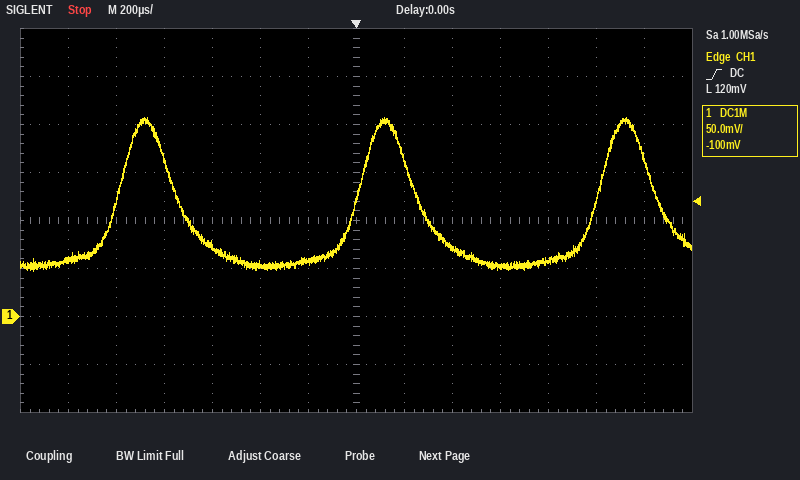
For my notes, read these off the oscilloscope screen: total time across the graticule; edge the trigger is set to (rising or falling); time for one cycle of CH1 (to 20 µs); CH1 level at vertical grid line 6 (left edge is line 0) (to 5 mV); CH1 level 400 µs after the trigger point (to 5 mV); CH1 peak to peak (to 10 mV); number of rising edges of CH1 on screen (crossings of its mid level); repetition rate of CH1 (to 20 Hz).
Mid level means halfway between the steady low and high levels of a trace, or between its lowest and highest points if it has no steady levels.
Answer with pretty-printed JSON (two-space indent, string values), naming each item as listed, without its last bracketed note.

{
  "total time across the graticule": "2.8 ms",
  "edge the trigger is set to": "rising",
  "time for one cycle of CH1": "1.00 ms",
  "CH1 level at vertical grid line 6 (left edge is line 0)": "55 mV",
  "CH1 level 400 µs after the trigger point": "70 mV",
  "CH1 peak to peak": "160 mV",
  "number of rising edges of CH1 on screen": "3",
  "repetition rate of CH1": "1.00 kHz"
}
